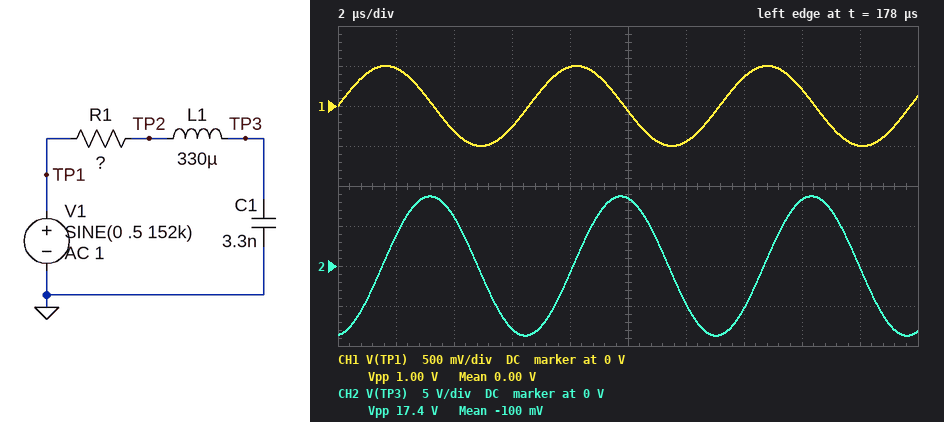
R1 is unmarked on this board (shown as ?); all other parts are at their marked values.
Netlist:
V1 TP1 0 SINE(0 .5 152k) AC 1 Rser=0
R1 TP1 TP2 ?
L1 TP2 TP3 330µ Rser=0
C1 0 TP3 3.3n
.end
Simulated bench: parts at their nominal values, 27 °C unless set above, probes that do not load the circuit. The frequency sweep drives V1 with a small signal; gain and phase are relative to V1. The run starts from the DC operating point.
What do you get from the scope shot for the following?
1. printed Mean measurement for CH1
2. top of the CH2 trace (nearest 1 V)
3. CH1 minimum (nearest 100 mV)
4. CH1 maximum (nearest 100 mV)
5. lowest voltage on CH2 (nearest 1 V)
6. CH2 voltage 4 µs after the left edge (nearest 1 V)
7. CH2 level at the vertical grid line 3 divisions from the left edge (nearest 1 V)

0.00 V
9 V
-500 mV
500 mV
-9 V
6 V
-8 V
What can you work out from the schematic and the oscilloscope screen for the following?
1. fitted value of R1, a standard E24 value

18 Ω
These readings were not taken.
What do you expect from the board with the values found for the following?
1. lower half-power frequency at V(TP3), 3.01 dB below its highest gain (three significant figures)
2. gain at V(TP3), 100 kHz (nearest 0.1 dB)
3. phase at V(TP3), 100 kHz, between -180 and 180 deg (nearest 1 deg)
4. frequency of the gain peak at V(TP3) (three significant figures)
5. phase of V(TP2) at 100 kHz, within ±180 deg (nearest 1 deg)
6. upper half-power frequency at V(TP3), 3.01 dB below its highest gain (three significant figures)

148 kHz
4.9 dB
-4 deg
152 kHz
-4 deg
157 kHz
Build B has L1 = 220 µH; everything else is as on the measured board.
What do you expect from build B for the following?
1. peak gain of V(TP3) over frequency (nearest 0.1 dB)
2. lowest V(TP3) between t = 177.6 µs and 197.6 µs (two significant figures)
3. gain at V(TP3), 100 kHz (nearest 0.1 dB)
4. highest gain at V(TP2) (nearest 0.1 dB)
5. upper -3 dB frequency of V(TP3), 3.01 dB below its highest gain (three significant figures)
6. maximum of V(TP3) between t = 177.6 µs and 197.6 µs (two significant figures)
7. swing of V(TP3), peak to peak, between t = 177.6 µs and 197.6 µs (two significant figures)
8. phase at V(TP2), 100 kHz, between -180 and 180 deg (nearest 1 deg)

23.1 dB
-1.5 V
2.9 dB
0 dB
193 kHz
1.5 V
2.9 V
-3 deg
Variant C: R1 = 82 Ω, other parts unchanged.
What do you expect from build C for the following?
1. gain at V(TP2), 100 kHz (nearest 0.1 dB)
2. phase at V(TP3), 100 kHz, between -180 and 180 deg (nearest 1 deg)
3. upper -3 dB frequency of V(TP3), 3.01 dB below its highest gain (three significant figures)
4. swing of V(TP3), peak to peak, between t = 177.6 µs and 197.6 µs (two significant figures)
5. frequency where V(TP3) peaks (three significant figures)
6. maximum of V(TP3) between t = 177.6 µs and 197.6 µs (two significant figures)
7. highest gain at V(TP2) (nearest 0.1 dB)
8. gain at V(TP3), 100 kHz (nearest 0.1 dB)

-0.4 dB
-17 deg
169 kHz
3.9 V
150 kHz
1.9 V
0 dB
4.5 dB
